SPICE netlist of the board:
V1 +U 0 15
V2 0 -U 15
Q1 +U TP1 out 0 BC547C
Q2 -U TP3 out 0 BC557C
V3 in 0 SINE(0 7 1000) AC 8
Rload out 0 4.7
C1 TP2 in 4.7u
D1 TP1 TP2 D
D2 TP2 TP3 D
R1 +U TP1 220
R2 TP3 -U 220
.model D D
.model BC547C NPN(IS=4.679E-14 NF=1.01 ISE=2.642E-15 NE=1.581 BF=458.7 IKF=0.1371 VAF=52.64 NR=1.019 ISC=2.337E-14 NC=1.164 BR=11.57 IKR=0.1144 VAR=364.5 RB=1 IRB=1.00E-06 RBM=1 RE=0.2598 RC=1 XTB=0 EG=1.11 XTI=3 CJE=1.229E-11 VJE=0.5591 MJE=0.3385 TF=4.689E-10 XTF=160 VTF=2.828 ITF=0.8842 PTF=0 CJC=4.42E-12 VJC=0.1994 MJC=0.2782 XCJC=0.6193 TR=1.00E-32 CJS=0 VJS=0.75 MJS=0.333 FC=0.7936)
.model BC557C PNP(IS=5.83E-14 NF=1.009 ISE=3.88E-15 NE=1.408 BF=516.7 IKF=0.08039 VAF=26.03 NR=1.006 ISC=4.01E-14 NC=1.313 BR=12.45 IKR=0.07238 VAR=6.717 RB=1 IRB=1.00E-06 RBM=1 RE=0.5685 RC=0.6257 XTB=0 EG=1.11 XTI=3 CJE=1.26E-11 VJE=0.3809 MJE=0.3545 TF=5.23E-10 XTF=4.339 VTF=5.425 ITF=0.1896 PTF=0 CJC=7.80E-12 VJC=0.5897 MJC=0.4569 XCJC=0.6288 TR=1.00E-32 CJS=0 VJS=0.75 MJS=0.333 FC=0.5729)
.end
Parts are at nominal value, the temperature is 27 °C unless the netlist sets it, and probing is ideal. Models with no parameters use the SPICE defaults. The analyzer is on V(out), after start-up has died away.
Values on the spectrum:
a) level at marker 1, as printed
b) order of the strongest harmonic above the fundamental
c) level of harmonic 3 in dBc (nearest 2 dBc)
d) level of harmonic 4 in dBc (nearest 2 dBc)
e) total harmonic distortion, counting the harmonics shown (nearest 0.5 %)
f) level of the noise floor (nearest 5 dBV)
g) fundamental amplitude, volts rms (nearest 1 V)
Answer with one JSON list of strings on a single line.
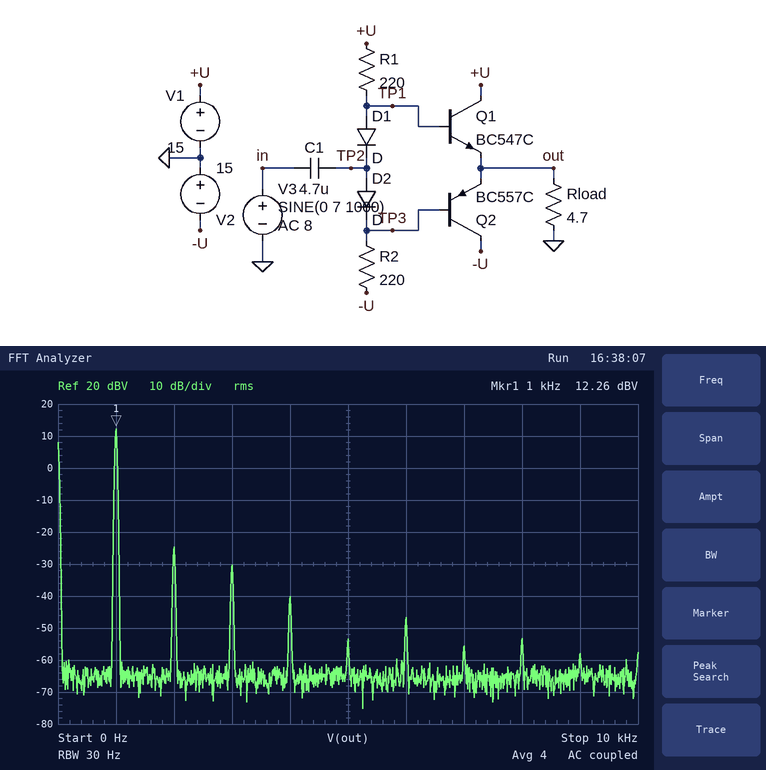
["12.26 dBV", "2", "-42 dBc", "-52 dBc", "1.5 %", "-65 dBV", "4 V"]
